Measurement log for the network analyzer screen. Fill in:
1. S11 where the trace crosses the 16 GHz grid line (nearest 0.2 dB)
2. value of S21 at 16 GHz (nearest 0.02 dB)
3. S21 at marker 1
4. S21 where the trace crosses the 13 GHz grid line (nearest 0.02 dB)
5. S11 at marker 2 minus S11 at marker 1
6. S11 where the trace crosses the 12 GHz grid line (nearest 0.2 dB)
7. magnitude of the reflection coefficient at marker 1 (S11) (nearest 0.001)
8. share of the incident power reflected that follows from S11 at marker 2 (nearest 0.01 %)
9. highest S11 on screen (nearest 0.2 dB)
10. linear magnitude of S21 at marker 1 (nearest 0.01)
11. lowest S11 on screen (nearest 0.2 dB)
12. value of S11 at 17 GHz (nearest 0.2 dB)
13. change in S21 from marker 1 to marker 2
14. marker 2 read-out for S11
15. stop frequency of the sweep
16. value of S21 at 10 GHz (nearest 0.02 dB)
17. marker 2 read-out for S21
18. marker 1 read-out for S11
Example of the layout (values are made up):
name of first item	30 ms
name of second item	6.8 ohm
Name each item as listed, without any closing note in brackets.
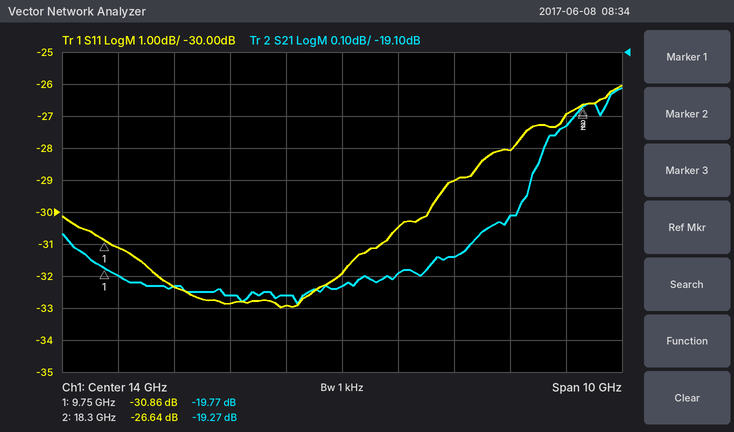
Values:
S11 where the trace crosses the 16 GHz grid line	-29.0 dB
value of S21 at 16 GHz	-19.74 dB
S21 at marker 1	-19.77 dB
S21 where the trace crosses the 13 GHz grid line	-19.86 dB
S11 at marker 2 minus S11 at marker 1	4.22 dB
S11 where the trace crosses the 12 GHz grid line	-32.8 dB
magnitude of the reflection coefficient at marker 1 (S11)	0.029
share of the incident power reflected that follows from S11 at marker 2	0.22 %
highest S11 on screen	-26.0 dB
linear magnitude of S21 at marker 1	0.10
lowest S11 on screen	-33.0 dB
value of S11 at 17 GHz	-28.0 dB
change in S21 from marker 1 to marker 2	0.50 dB
marker 2 read-out for S11	-26.64 dB
stop frequency of the sweep	19 GHz
value of S21 at 10 GHz	-19.80 dB
marker 2 read-out for S21	-19.27 dB
marker 1 read-out for S11	-30.86 dB
